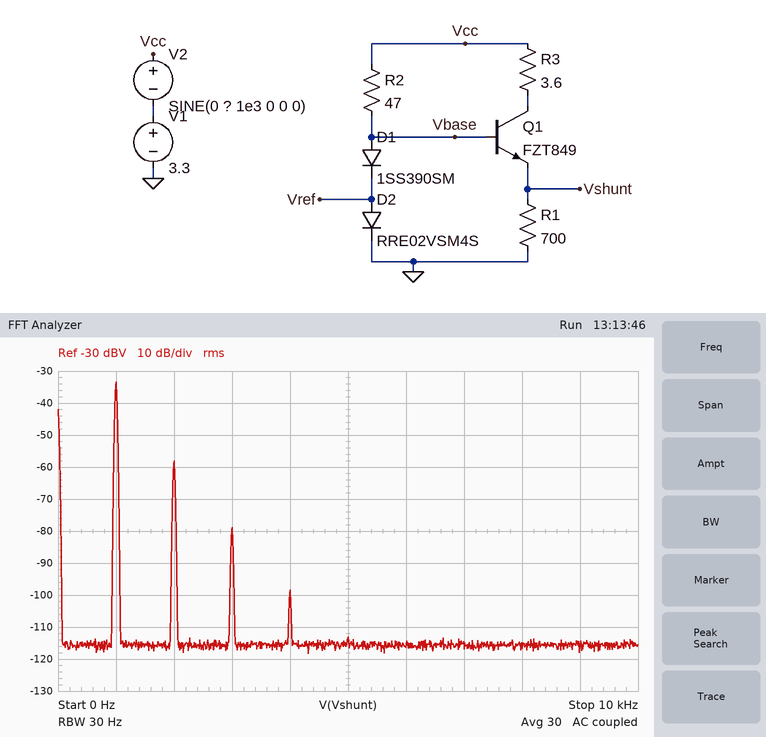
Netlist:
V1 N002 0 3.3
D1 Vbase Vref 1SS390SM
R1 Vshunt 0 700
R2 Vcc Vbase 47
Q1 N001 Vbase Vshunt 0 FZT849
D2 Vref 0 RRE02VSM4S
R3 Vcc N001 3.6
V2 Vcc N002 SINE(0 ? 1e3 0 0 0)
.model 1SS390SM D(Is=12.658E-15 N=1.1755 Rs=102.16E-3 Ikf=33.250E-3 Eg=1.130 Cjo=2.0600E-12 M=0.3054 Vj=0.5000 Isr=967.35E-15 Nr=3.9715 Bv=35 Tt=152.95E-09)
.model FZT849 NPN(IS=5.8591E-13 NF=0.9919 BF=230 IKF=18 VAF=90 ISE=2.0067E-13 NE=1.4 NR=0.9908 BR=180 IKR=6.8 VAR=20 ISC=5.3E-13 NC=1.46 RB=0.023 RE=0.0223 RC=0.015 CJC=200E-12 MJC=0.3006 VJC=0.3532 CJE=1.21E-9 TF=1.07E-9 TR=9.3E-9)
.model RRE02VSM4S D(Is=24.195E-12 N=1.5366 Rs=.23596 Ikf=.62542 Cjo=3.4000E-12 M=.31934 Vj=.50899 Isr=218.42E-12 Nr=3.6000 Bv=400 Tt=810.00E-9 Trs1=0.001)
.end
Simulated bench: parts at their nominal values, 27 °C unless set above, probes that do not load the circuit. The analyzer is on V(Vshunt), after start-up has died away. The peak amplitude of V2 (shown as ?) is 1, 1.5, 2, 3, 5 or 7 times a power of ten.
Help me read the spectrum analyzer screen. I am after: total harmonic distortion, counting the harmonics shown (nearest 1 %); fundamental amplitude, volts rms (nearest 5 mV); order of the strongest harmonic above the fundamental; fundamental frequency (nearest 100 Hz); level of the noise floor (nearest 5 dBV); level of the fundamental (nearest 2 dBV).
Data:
6 %
20 mV
2
1.0 kHz
-115 dBV
-34 dBV
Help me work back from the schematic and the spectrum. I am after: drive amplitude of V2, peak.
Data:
500 mV
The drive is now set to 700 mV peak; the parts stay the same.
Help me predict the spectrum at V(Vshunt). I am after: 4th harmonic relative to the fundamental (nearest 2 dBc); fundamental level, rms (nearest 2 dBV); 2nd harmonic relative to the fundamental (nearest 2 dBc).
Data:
-56 dBc
-30 dBV
-22 dBc
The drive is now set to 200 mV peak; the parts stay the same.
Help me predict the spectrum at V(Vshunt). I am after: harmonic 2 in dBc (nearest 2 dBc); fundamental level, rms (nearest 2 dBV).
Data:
-32 dBc
-42 dBV
